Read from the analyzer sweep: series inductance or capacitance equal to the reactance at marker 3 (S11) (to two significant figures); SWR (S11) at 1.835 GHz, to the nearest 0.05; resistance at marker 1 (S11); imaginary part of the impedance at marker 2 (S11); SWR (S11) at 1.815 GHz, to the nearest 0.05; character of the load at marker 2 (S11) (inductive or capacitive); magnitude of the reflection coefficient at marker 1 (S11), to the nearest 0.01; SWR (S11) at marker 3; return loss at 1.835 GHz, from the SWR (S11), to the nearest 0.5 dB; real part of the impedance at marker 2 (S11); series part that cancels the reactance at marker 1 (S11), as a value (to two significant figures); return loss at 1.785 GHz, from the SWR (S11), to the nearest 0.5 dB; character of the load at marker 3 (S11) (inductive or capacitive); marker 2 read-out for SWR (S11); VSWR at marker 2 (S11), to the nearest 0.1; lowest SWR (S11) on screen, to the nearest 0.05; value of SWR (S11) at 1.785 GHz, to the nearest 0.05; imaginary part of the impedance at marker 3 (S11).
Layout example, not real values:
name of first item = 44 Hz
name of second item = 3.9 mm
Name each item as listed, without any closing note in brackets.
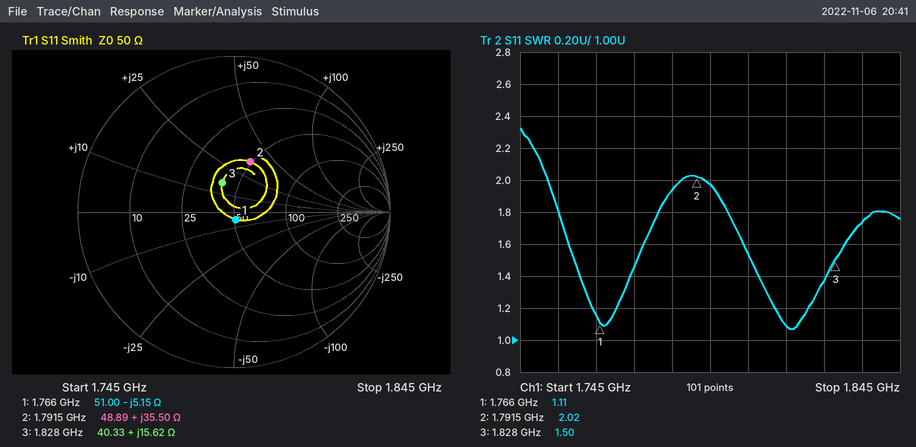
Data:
series inductance or capacitance equal to the reactance at marker 3 (S11) = 1.4 nH
SWR (S11) at 1.835 GHz, to the nearest 0.05 = 1.75
resistance at marker 1 = 51.00 Ω
imaginary part of the impedance at marker 2 = +35.50 Ω
SWR (S11) at 1.815 GHz, to the nearest 0.05 = 1.10
character of the load at marker 2 (S11) = inductive
magnitude of the reflection coefficient at marker 1 (S11), to the nearest 0.01 = 0.05
SWR (S11) at marker 3 = 1.50
return loss at 1.835 GHz, from the SWR (S11), to the nearest 0.5 dB = 11.5 dB
real part of the impedance at marker 2 = 48.89 Ω
series part that cancels the reactance at marker 1 (S11), as a value = 460 pH
return loss at 1.785 GHz, from the SWR (S11), to the nearest 0.5 dB = 10.0 dB
character of the load at marker 3 (S11) = inductive
marker 2 read-out for SWR = 2.02
VSWR at marker 2 (S11), to the nearest 0.1 = 2.0
lowest SWR (S11) on screen, to the nearest 0.05 = 1.05
value of SWR (S11) at 1.785 GHz, to the nearest 0.05 = 1.95
imaginary part of the impedance at marker 3 = +15.62 Ω
